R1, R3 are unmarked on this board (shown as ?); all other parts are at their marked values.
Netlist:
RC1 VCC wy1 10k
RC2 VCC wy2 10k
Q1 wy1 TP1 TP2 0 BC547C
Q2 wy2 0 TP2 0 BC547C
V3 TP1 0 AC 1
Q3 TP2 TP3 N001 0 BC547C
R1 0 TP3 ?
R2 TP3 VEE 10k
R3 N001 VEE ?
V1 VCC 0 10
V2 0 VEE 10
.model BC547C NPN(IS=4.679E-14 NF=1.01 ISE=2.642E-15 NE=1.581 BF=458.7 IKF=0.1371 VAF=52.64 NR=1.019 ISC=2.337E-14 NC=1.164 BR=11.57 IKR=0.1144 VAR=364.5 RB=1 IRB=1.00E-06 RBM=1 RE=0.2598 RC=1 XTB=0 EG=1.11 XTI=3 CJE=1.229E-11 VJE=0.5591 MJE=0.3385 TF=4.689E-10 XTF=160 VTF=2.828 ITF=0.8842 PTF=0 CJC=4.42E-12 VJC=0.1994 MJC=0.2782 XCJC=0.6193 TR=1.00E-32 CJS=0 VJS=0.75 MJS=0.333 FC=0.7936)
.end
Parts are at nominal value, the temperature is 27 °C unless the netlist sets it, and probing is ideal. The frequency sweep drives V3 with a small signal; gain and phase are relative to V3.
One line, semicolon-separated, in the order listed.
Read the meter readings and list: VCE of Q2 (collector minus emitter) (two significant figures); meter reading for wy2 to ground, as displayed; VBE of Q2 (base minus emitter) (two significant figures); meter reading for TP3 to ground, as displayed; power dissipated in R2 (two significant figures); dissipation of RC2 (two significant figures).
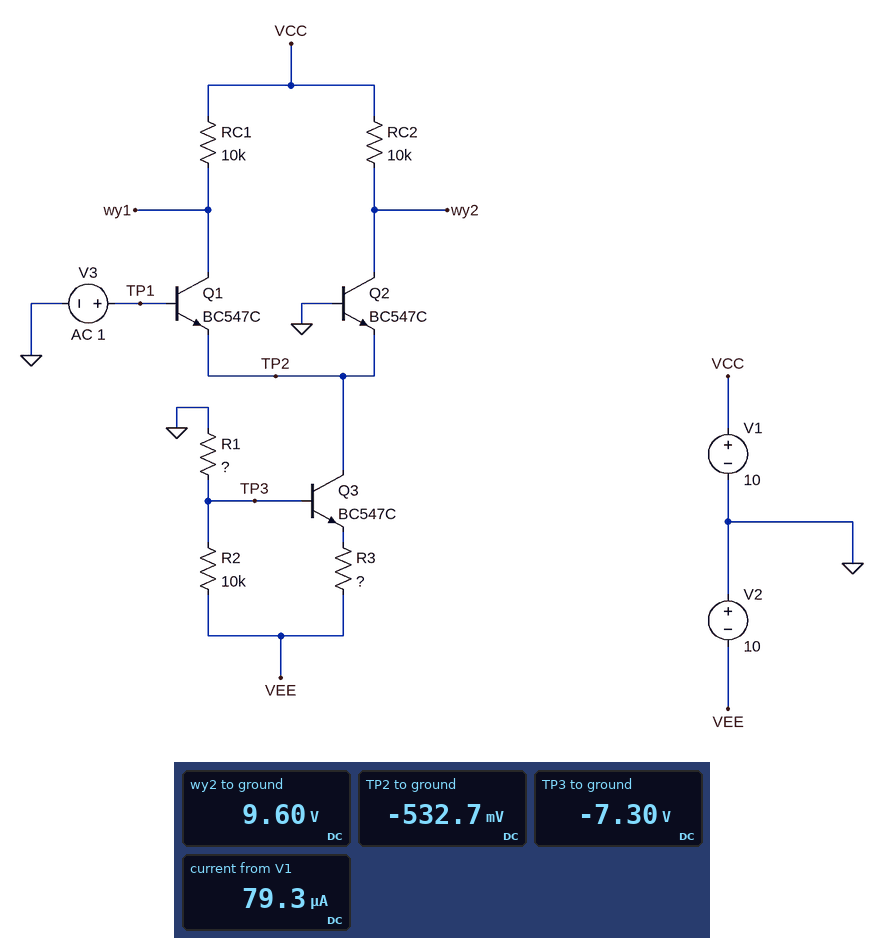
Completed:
10 V; 9.60 V; 530 mV; -7.30 V; 730 µW; 16 µW
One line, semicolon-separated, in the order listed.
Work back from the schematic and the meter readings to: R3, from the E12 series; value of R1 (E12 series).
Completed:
27 kΩ; 27 kΩ
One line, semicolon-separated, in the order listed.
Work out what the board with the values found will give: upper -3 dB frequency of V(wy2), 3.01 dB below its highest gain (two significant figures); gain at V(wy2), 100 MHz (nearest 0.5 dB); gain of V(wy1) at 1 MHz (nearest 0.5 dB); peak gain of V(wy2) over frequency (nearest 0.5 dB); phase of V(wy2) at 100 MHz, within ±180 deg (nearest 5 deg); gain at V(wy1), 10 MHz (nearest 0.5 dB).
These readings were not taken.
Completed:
10 MHz; -2.0 dB; 17.5 dB; 17.5 dB; -85 deg; 15.0 dB
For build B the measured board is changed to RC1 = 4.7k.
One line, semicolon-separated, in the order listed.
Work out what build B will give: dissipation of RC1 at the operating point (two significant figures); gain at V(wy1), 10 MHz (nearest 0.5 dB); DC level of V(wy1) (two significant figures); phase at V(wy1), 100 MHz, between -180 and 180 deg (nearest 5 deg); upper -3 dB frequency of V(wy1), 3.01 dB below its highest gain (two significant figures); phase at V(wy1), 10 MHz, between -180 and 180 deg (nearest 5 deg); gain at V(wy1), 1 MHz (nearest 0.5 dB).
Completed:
7.4 µW; 10.5 dB; 9.8 V; 50 deg; 26 MHz; 150 deg; 11.0 dB
